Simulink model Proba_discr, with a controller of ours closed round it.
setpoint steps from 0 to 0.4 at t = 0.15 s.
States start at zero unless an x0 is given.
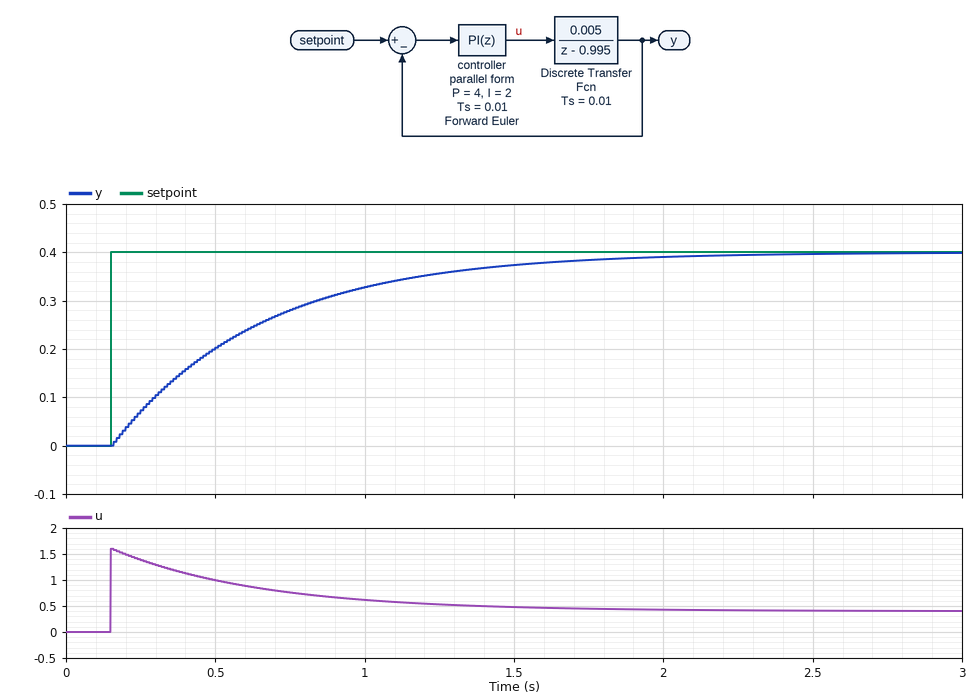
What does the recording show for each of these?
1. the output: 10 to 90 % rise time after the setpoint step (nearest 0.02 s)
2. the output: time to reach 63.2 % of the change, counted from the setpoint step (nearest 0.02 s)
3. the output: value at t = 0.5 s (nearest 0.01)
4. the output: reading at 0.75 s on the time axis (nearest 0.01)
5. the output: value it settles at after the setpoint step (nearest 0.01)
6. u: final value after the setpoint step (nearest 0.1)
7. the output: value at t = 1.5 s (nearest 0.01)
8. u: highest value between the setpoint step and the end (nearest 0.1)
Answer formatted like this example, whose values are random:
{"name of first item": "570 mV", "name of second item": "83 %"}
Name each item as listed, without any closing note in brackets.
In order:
{"the output: 10 to 90 % rise time after the setpoint step": "1.08 s", "the output: time to reach 63.2 % of the change, counted from the setpoint step": "0.50 s", "the output: value at t = 0.5 s": "0.20", "the output: reading at 0.75 s on the time axis": "0.28", "the output: value it settles at after the setpoint step": "0.40", "u: final value after the setpoint step": "0.4", "the output: value at t = 1.5 s": "0.37", "u: highest value between the setpoint step and the end": "1.6"}
